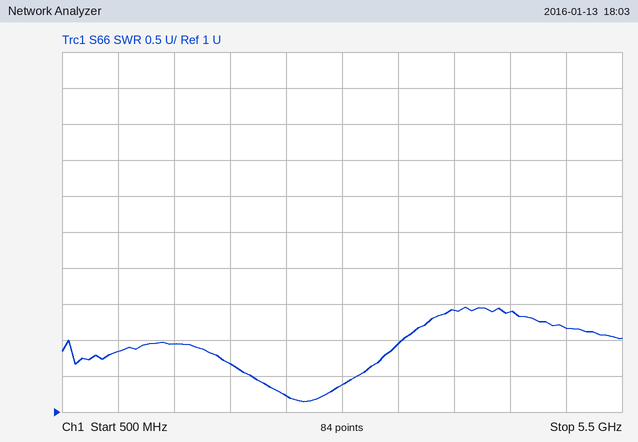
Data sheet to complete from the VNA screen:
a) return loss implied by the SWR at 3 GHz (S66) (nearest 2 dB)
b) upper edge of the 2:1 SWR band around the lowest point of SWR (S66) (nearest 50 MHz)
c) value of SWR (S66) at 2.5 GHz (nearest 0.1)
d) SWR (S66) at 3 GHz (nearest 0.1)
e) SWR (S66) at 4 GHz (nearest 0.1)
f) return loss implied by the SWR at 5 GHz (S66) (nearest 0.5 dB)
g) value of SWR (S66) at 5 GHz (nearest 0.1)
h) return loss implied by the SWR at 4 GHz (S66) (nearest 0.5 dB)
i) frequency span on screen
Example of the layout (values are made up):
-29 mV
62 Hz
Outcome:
16 dB
3.55 GHz
1.2
1.4
2.4
8.5 dB
2.2
7.5 dB
5 GHz
